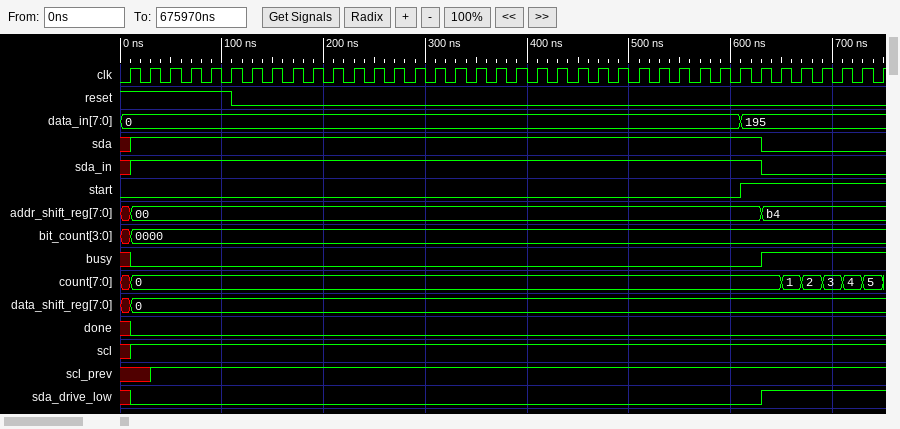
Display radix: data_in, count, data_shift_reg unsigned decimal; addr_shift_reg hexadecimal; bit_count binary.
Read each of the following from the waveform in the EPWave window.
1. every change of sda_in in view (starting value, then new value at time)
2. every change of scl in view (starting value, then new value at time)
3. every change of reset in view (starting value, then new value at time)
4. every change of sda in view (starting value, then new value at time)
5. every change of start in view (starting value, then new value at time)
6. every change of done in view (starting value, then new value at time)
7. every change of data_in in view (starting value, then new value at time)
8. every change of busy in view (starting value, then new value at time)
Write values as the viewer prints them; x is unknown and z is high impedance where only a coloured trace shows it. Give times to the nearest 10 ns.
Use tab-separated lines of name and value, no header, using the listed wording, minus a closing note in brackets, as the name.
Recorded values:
every change of sda_in in view	x, 1 at 10 ns, 0 at 630 ns
every change of scl in view	x, 1 at 10 ns
every change of reset in view	1, 0 at 110 ns
every change of sda in view	x, 1 at 10 ns, 0 at 630 ns
every change of start in view	0, 1 at 610 ns
every change of done in view	x, 0 at 10 ns
every change of data_in in view	0, 195 at 610 ns
every change of busy in view	x, 0 at 10 ns, 1 at 630 ns
